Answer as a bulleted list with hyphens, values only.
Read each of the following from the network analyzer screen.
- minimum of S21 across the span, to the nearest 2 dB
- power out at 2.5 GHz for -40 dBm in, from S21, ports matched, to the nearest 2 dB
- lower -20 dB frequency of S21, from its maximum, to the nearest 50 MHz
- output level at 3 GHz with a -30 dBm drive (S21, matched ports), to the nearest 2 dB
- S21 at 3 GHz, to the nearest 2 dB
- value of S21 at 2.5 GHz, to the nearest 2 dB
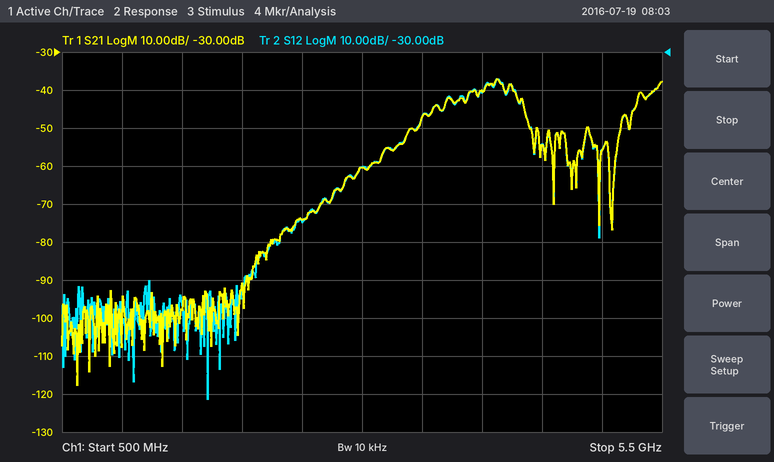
- -118 dB
- -114 dBm
- 3.15 GHz
- -90 dBm
- -60 dB
- -74 dB
